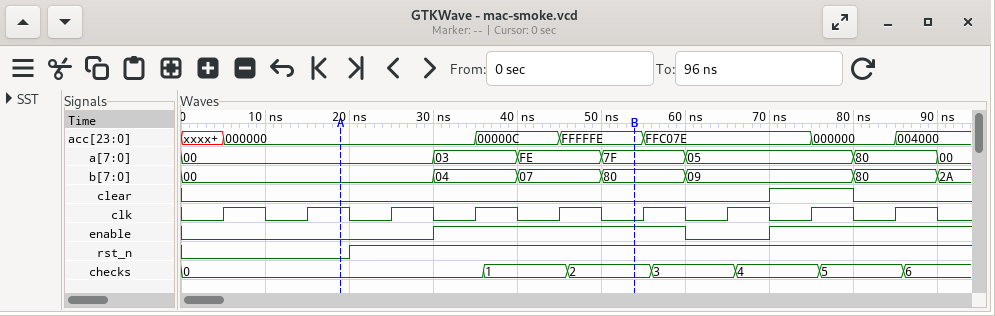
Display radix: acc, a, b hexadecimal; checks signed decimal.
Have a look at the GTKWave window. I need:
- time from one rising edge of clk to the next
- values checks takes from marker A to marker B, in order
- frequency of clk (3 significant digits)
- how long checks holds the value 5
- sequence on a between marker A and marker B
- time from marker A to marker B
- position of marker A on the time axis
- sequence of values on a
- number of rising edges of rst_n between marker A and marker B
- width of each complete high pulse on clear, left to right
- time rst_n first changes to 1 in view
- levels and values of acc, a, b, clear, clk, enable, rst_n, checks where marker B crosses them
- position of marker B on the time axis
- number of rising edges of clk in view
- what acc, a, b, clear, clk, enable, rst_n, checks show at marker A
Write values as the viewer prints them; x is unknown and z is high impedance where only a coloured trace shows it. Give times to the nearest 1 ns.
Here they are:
10 ns
0, 1, 2
100 MHz
10 ns
00, 03, FE, 7F
35 ns
19 ns
00, 03, FE, 7F, 05, 80, 00
1
10 ns
20 ns
acc=FFFFFE, a=7F, b=80, clear=0, clk=0, enable=1, rst_n=1, checks=2
54 ns
9
acc=000000, a=00, b=00, clear=0, clk=1, enable=0, rst_n=0, checks=0
